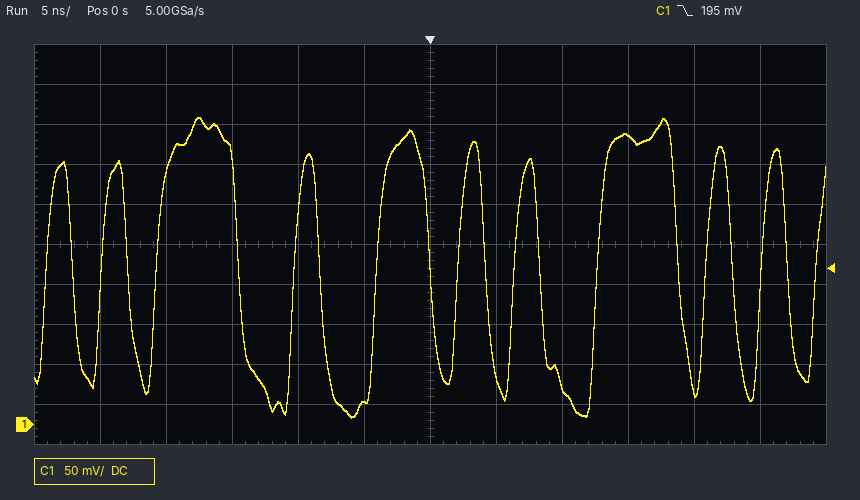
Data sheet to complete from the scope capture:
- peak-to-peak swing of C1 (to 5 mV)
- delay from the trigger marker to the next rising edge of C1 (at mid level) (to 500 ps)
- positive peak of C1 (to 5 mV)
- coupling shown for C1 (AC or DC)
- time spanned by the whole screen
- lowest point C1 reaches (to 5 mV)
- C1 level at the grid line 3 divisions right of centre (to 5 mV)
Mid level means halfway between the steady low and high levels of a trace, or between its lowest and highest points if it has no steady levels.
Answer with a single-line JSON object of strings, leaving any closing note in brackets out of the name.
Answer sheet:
{"peak-to-peak swing of C1": "375 mV", "delay from the trigger marker to the next rising edge of C1 (at mid level)": "2.0 ns", "positive peak of C1": "385 mV", "coupling shown for C1": "DC", "time spanned by the whole screen": "60 ns", "lowest point C1 reaches": "10 mV", "C1 level at the grid line 3 divisions right of centre": "360 mV"}
